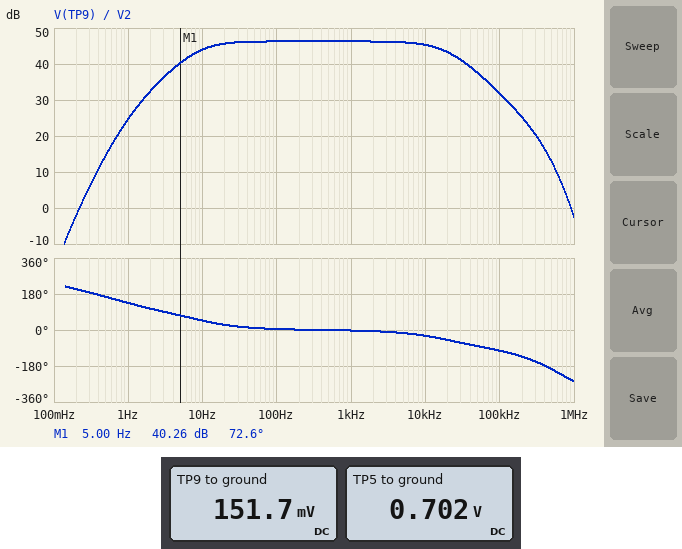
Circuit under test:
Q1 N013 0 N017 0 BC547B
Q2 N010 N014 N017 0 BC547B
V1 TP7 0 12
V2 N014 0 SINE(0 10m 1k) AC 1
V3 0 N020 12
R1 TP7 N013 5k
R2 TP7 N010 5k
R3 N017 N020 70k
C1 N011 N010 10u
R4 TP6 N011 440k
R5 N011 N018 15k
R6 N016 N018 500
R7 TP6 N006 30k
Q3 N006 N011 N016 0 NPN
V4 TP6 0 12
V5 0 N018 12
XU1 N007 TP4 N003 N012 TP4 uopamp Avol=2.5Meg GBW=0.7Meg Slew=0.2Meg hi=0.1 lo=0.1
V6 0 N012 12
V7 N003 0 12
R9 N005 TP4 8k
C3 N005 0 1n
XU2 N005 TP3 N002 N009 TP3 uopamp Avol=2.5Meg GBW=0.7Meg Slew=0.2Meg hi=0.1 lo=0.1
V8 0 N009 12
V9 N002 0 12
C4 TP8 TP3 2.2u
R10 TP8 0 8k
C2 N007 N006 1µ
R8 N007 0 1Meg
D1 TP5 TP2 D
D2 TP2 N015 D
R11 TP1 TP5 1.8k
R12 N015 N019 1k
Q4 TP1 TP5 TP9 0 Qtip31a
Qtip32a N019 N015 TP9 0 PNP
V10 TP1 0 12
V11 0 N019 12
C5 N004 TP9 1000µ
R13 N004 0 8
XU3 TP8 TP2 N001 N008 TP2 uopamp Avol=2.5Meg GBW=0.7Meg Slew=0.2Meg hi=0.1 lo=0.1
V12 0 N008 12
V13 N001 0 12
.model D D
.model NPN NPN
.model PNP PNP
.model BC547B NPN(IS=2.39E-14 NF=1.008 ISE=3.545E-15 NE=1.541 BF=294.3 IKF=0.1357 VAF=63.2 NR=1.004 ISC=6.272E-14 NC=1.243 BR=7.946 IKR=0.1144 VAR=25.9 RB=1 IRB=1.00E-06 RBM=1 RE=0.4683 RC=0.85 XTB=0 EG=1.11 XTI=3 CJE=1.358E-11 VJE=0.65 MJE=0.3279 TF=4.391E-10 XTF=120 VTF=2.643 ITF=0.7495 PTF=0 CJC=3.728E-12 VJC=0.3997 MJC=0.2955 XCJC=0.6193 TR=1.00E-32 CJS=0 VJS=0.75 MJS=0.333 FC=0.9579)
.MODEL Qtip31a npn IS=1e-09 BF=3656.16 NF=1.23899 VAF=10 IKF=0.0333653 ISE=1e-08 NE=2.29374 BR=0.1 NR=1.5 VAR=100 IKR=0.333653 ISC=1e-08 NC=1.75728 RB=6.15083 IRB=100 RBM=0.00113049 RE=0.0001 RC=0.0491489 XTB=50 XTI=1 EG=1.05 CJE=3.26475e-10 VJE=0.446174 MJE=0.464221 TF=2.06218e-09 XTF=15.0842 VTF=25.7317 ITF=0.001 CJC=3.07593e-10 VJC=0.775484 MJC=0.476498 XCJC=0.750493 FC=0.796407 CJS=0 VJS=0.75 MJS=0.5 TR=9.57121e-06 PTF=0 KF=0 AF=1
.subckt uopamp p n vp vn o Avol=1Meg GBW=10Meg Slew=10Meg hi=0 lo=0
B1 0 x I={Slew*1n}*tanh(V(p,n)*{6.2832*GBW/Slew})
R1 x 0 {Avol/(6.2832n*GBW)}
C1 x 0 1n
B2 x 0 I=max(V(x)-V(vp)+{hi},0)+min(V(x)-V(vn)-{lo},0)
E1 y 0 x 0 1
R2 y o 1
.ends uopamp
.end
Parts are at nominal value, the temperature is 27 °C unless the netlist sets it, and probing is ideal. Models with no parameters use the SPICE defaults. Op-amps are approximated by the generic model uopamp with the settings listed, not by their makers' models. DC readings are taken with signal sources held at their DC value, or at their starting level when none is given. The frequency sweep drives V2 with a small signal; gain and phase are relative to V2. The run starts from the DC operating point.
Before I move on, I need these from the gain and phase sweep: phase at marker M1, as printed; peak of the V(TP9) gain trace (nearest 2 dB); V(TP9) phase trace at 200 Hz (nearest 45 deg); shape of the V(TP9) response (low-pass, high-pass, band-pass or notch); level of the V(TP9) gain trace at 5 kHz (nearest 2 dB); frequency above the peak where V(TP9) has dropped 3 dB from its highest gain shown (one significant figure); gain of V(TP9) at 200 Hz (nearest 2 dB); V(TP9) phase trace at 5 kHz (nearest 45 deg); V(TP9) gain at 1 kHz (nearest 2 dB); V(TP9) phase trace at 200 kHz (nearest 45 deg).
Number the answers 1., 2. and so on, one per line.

1. 72.6 deg
2. 46 dB
3. 0 deg
4. band-pass
5. 46 dB
6. 20 kHz
7. 46 dB
8. 0 deg
9. 46 dB
10. -135 deg
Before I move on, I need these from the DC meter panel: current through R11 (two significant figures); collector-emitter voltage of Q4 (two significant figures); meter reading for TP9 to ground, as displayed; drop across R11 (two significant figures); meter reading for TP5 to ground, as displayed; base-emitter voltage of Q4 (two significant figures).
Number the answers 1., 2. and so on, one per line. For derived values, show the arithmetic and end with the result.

1. (12 V - 702 mV) / 1.8 kΩ = 6.3 mA
2. 12 V - 151.7 mV = 12 V
3. 151.7 mV
4. 12 V - 702 mV = 11 V
5. 0.702 V
6. 702 mV - 151.7 mV = 550 mV
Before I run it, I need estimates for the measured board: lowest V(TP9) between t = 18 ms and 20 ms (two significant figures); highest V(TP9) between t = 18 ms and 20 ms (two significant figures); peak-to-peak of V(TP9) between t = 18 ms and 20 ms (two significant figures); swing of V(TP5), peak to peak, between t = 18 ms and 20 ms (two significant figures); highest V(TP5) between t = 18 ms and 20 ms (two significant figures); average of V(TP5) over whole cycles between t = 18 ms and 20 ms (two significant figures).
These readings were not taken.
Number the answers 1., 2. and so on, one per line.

1. -2.0 V
2. 2.0 V
3. 4.0 V
4. 4.2 V
5. 2.6 V
6. 660 mV
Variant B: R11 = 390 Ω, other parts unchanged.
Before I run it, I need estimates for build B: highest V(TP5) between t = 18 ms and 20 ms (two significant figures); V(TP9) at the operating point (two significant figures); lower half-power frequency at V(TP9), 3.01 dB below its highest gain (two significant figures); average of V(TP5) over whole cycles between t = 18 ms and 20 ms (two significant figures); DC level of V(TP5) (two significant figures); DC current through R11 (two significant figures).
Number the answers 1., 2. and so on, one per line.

1. 2.7 V
2. 170 mV
3. 8.7 Hz
4. 700 mV
5. 740 mV
6. 29 mA
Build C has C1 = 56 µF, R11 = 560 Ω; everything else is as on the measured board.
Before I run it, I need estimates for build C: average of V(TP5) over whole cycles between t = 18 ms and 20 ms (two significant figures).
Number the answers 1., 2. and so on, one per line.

1. 690 mV
